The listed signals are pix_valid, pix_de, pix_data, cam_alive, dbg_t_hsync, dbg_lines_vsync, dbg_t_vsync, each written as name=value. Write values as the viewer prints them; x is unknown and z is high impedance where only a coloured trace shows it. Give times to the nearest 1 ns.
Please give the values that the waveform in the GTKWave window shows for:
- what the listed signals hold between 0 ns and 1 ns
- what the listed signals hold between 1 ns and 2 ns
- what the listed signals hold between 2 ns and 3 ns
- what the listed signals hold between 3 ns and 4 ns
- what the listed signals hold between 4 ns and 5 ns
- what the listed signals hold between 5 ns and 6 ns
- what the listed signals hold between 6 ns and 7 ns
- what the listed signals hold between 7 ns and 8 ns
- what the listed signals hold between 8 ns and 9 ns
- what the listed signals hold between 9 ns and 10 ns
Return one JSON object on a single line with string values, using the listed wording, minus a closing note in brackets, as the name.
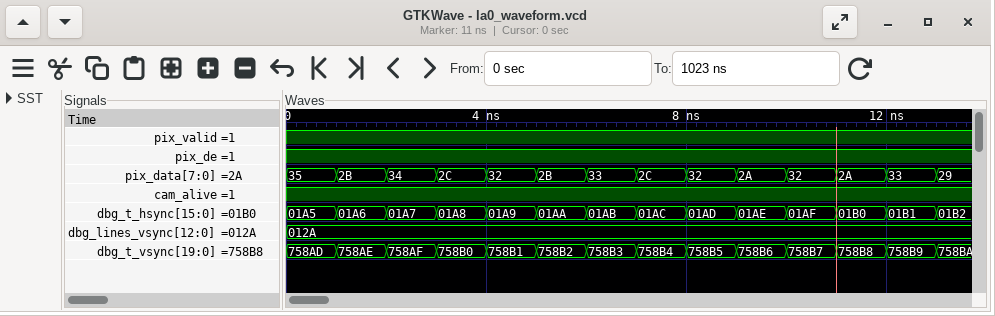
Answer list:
{"what the listed signals hold between 0 ns and 1 ns": "pix_valid=1, pix_de=1, pix_data=35, cam_alive=1, dbg_t_hsync=01A5, dbg_lines_vsync=012A, dbg_t_vsync=758AD", "what the listed signals hold between 1 ns and 2 ns": "pix_valid=1, pix_de=1, pix_data=2B, cam_alive=1, dbg_t_hsync=01A6, dbg_lines_vsync=012A, dbg_t_vsync=758AE", "what the listed signals hold between 2 ns and 3 ns": "pix_valid=1, pix_de=1, pix_data=34, cam_alive=1, dbg_t_hsync=01A7, dbg_lines_vsync=012A, dbg_t_vsync=758AF", "what the listed signals hold between 3 ns and 4 ns": "pix_valid=1, pix_de=1, pix_data=2C, cam_alive=1, dbg_t_hsync=01A8, dbg_lines_vsync=012A, dbg_t_vsync=758B0", "what the listed signals hold between 4 ns and 5 ns": "pix_valid=1, pix_de=1, pix_data=32, cam_alive=1, dbg_t_hsync=01A9, dbg_lines_vsync=012A, dbg_t_vsync=758B1", "what the listed signals hold between 5 ns and 6 ns": "pix_valid=1, pix_de=1, pix_data=2B, cam_alive=1, dbg_t_hsync=01AA, dbg_lines_vsync=012A, dbg_t_vsync=758B2", "what the listed signals hold between 6 ns and 7 ns": "pix_valid=1, pix_de=1, pix_data=33, cam_alive=1, dbg_t_hsync=01AB, dbg_lines_vsync=012A, dbg_t_vsync=758B3", "what the listed signals hold between 7 ns and 8 ns": "pix_valid=1, pix_de=1, pix_data=2C, cam_alive=1, dbg_t_hsync=01AC, dbg_lines_vsync=012A, dbg_t_vsync=758B4", "what the listed signals hold between 8 ns and 9 ns": "pix_valid=1, pix_de=1, pix_data=32, cam_alive=1, dbg_t_hsync=01AD, dbg_lines_vsync=012A, dbg_t_vsync=758B5", "what the listed signals hold between 9 ns and 10 ns": "pix_valid=1, pix_de=1, pix_data=2A, cam_alive=1, dbg_t_hsync=01AE, dbg_lines_vsync=012A, dbg_t_vsync=758B6"}
